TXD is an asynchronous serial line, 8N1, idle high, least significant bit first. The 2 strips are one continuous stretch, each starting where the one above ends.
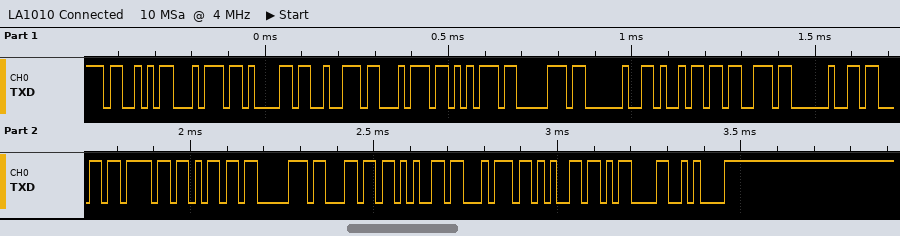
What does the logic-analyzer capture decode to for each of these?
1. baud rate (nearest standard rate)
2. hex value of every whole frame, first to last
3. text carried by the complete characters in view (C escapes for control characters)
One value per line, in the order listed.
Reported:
57600 baud
0x53 0x74 0x61 0x72 0x74 0x75 0x70 0x20 0x69 0x73 0x20 0x63 0x6F 0x6D 0x70 0x6C 0x65 0x74 0x65 0x0D 0x0A
"Startup is complete\r\n"
